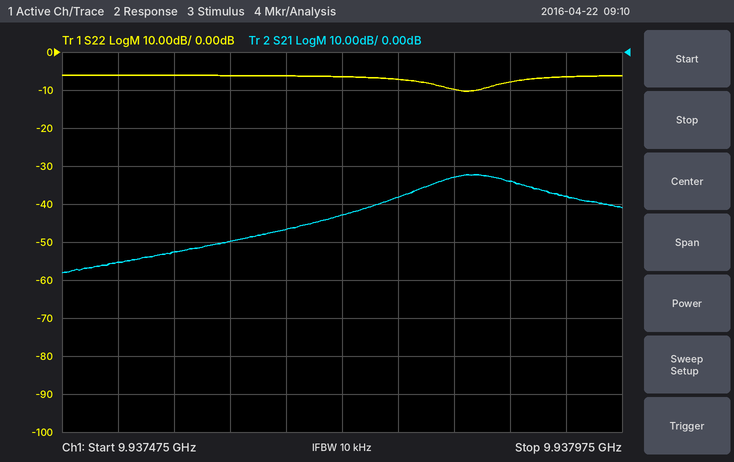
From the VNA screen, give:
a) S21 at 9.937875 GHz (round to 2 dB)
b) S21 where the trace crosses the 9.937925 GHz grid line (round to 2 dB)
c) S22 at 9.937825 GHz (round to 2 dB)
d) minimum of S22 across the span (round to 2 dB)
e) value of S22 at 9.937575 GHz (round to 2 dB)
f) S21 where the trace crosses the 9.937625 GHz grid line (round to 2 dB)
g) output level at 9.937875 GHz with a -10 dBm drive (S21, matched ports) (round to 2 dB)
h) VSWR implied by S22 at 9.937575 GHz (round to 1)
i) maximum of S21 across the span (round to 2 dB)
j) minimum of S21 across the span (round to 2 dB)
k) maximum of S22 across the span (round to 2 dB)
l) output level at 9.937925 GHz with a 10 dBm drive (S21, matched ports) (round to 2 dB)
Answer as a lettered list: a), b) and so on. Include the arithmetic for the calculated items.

a) -34 dB
b) -38 dB
c) -10 dB
d) -10 dB
e) -6 dB
f) -50 dB
g) -10 dBm + (-34 dB) = -44 dBm
h) |Γ| = 10^(-6/20) = 0.5012; VSWR = (1 + 0.5012)/(1 − 0.5012) ≈ 3
i) -32 dB
j) -58 dB
k) -6 dB
l) 10 dBm + (-38 dB) = -28 dBm
